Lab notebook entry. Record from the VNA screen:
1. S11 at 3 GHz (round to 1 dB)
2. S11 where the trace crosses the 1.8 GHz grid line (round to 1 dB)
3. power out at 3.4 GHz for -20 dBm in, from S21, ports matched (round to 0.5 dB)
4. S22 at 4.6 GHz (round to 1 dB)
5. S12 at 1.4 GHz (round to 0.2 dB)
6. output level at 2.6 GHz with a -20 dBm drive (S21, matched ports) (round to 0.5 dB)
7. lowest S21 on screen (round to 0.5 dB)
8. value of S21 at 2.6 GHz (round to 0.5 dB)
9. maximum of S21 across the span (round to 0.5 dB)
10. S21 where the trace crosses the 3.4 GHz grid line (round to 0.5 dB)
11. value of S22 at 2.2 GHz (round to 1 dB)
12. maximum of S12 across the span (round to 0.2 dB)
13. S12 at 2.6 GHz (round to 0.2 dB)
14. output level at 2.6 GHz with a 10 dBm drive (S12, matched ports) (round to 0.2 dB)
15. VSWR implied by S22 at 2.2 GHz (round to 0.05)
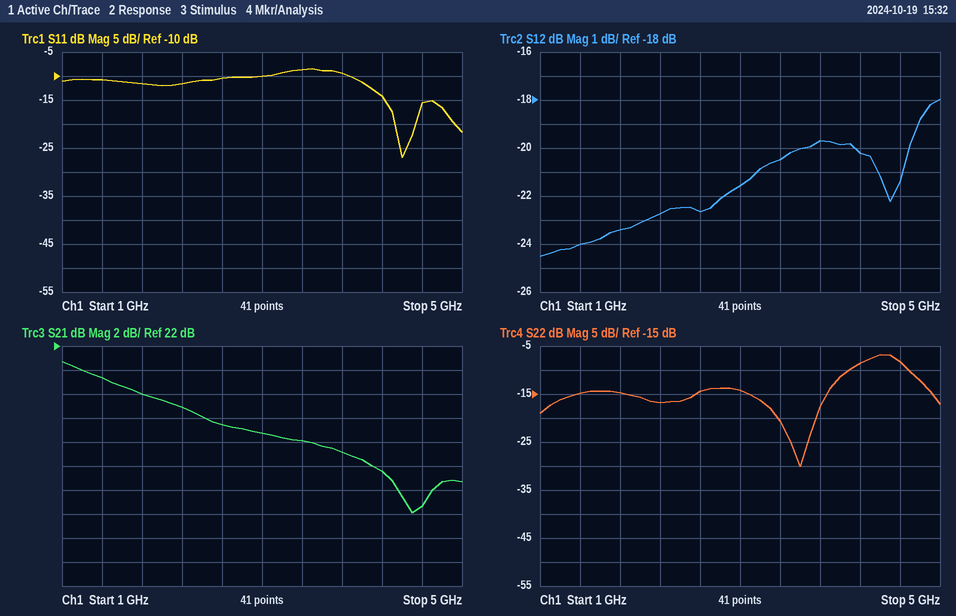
-10 dB
-12 dB
-6.0 dBm
-8 dB
-24.0 dB
-4.5 dBm
8.0 dB
15.5 dB
20.5 dB
14.0 dB
-17 dB
-18.0 dB
-22.6 dB
-12.6 dBm
1.35
